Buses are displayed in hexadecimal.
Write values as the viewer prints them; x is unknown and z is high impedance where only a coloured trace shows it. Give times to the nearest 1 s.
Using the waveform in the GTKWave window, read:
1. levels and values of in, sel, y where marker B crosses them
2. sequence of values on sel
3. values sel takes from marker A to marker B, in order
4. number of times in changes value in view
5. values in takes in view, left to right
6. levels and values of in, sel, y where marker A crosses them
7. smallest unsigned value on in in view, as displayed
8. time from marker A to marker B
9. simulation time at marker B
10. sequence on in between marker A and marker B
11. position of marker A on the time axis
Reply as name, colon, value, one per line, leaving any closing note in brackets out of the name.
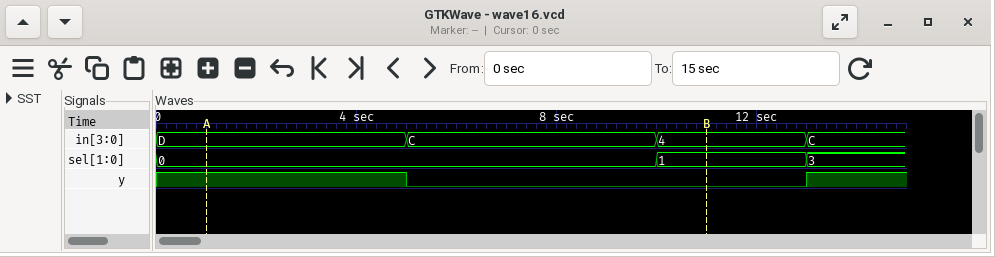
levels and values of in, sel, y where marker B crosses them: in=4, sel=1, y=0
sequence of values on sel: 0, 1, 3
values sel takes from marker A to marker B, in order: 0, 1
number of times in changes value in view: 3
values in takes in view, left to right: D, C, 4, C
levels and values of in, sel, y where marker A crosses them: in=D, sel=0, y=1
smallest unsigned value on in in view, as displayed: 4
time from marker A to marker B: 10 s
simulation time at marker B: 11 s
sequence on in between marker A and marker B: D, C, 4
position of marker A on the time axis: 1 s
